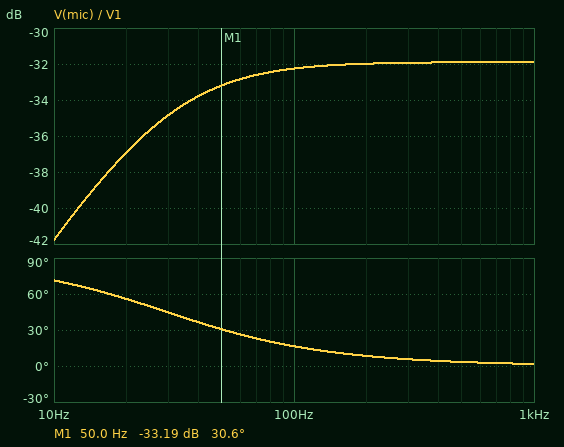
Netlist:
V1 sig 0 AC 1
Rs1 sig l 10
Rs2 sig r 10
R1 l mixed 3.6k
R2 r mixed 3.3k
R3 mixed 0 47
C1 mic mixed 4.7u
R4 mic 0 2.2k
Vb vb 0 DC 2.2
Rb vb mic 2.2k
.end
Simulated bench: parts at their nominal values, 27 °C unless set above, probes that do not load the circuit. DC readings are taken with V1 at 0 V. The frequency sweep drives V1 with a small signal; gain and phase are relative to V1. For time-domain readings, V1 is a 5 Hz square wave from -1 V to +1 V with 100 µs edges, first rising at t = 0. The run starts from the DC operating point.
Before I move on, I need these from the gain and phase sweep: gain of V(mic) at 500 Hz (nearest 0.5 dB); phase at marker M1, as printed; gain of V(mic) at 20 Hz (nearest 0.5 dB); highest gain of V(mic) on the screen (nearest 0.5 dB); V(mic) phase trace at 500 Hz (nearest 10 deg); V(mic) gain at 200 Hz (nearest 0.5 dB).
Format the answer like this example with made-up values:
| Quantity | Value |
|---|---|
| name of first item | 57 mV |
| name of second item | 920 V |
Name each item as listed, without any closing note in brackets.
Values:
| Quantity | Value |
|---|---|
| gain of V(mic) at 500 Hz | -32.0 dB |
| phase at marker M1, as printed | 30.6 deg |
| gain of V(mic) at 20 Hz | -37.0 dB |
| highest gain of V(mic) on the screen | -32.0 dB |
| V(mic) phase trace at 500 Hz | 0 deg |
| V(mic) gain at 200 Hz | -32.0 dB |
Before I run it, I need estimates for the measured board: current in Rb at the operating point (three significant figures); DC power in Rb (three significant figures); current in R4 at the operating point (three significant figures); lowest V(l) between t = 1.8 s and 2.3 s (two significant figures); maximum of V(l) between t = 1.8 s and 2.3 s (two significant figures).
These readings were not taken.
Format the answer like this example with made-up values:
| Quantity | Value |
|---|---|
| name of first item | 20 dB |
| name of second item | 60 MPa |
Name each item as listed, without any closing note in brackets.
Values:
| Quantity | Value |
|---|---|
| current in Rb at the operating point | 500 µA |
| DC power in Rb | 550 µW |
| current in R4 at the operating point | 500 µA |
| lowest V(l) between t = 1.8 s and 2.3 s | -1.0 V |
| maximum of V(l) between t = 1.8 s and 2.3 s | 1.0 V |
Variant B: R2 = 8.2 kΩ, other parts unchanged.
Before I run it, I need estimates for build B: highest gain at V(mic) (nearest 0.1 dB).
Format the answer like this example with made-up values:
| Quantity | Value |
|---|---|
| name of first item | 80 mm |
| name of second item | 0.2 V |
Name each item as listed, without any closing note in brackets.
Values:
| Quantity | Value |
|---|---|
| highest gain at V(mic) | -35.1 dB |
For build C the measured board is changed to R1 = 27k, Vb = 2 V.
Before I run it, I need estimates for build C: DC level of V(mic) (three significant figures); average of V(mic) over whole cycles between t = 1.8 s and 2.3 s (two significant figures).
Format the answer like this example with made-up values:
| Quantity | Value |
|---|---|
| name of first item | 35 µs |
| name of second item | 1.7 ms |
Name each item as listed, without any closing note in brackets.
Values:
| Quantity | Value |
|---|---|
| DC level of V(mic) | 1.00 V |
| average of V(mic) over whole cycles between t = 1.8 s and 2.3 s | 1.0 V |
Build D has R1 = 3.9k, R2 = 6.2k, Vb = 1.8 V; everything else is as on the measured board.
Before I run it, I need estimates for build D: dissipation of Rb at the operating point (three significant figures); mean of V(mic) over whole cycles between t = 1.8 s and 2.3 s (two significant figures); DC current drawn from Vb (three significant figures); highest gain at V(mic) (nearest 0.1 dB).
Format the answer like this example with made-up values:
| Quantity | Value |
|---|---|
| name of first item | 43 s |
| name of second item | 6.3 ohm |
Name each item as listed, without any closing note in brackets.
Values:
| Quantity | Value |
|---|---|
| dissipation of Rb at the operating point | 368 µW |
| mean of V(mic) over whole cycles between t = 1.8 s and 2.3 s | 900 mV |
| DC current drawn from Vb | 409 µA |
| highest gain at V(mic) | -34.7 dB |
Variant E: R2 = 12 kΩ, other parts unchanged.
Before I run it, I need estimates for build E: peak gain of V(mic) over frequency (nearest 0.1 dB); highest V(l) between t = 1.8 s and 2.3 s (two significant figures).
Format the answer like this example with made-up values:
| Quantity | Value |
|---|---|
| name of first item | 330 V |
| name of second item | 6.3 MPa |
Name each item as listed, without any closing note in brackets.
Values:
| Quantity | Value |
|---|---|
| peak gain of V(mic) over frequency | -35.9 dB |
| highest V(l) between t = 1.8 s and 2.3 s | 1.0 V |
